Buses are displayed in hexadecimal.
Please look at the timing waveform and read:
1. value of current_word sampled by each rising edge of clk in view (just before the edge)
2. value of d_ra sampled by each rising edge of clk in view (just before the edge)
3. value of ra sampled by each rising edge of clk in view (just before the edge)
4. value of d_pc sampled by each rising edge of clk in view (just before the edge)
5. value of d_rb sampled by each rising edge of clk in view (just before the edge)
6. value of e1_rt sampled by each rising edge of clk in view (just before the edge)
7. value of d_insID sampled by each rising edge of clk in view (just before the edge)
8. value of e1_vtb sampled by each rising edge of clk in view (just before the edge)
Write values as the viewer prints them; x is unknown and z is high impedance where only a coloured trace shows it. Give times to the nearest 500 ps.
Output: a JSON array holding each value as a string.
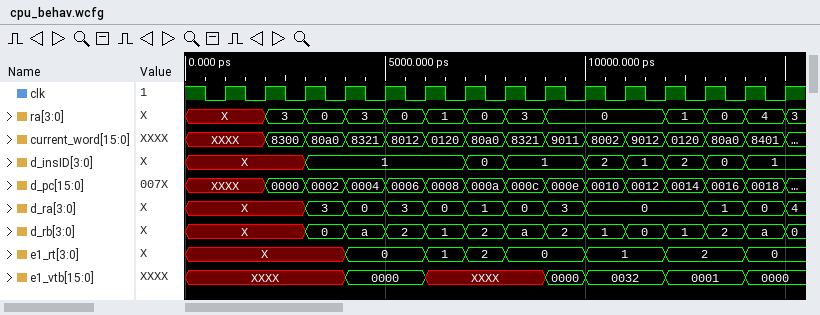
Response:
["XXXX, XXXX, 8300, 80a0, 8321, 8012, 0120, 80a0, 8321, 9011, 8002, 9012, 0120, 80a0, 8401", "X, X, X, 3, 0, 3, 0, 1, 0, 3, 0, 0, 0, 1, 0", "X, X, 3, 0, 3, 0, 1, 0, 3, 0, 0, 0, 1, 0, 4", "XXXX, XXXX, 0000, 0002, 0004, 0006, 0008, 000a, 000c, 000e, 0010, 0012, 0014, 0016, 0018", "X, X, X, 0, a, 2, 1, 2, a, 2, 1, 0, 1, 2, a", "X, X, X, X, 0, 0, 1, 2, 0, 0, 1, 1, 2, 2, 0", "X, X, X, 1, 1, 1, 1, 0, 1, 1, 2, 1, 2, 0, 1", "XXXX, XXXX, XXXX, XXXX, 0000, 0000, XXXX, XXXX, XXXX, 0000, 0032, 0032, 0001, 0001, 0000"]
